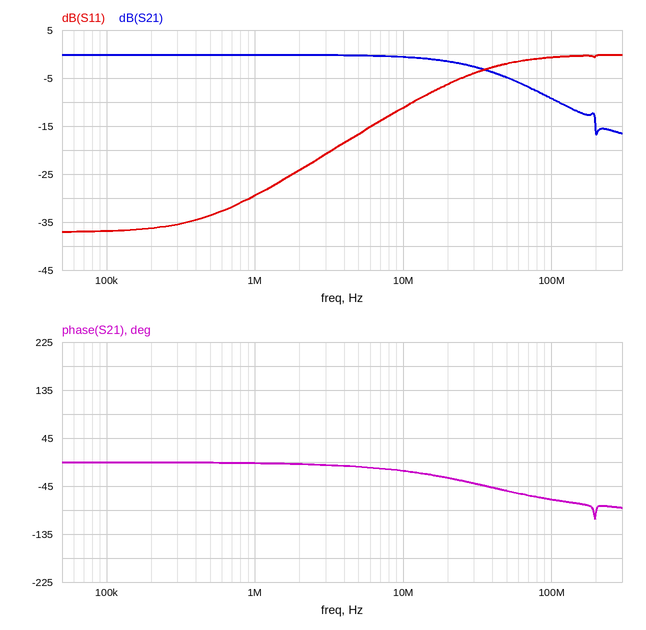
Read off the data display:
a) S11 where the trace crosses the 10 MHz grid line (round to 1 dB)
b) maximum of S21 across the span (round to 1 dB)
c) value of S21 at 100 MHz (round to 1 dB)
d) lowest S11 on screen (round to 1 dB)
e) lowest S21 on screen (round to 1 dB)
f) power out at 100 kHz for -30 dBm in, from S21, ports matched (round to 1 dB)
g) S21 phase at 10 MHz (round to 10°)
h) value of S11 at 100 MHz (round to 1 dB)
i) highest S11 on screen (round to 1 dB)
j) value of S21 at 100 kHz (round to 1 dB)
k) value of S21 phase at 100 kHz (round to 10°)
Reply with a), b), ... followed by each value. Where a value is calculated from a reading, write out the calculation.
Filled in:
a) -11 dB
b) 0 dB
c) -9 dB
d) -37 dB
e) -17 dB
f) -30 dBm + (0 dB) = -30 dBm
g) -20°
h) -1 dB
i) 0 dB
j) 0 dB
k) 0°
